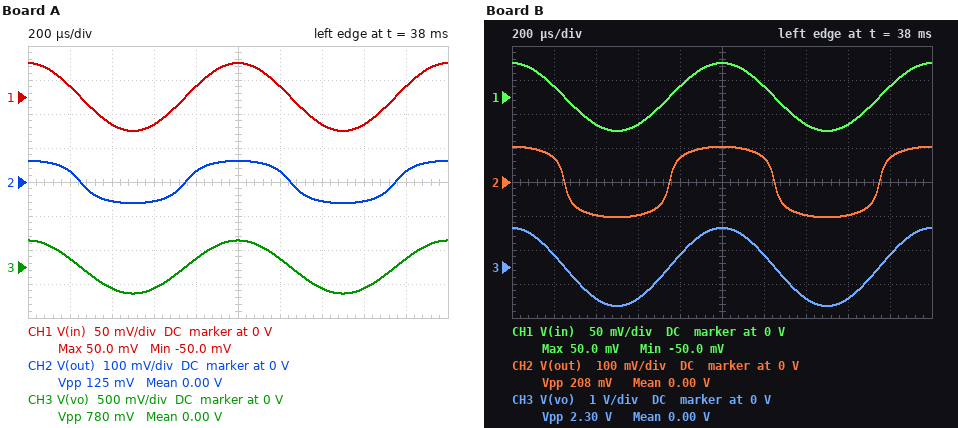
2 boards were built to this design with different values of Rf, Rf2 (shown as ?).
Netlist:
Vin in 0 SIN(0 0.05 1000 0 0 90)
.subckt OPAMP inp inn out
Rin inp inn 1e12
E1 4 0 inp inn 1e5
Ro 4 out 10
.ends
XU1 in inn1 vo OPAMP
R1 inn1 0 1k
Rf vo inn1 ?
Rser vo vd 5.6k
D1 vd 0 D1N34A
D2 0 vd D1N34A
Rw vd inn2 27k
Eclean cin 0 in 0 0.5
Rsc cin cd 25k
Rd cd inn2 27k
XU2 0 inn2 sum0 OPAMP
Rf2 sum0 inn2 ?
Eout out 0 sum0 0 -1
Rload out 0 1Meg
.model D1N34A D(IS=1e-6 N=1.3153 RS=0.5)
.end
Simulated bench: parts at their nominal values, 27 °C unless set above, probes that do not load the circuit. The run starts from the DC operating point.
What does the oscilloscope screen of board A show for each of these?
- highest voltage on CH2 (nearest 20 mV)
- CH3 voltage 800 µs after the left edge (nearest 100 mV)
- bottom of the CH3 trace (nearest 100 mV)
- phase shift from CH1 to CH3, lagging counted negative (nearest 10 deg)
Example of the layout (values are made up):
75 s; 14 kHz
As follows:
60 mV; 100 mV; -400 mV; 0 deg
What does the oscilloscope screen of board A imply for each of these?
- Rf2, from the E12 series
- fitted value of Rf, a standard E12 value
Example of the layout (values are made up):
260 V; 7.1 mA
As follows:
12 kΩ; 6.8 kΩ
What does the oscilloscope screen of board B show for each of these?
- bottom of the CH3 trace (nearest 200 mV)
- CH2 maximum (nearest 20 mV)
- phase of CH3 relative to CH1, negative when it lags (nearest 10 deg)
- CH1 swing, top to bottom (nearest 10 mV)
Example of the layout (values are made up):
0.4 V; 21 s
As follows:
-1.2 V; 100 mV; 0 deg; 100 mV
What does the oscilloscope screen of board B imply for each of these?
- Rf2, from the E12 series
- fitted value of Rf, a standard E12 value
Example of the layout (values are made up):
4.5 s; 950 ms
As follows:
15 kΩ; 22 kΩ
